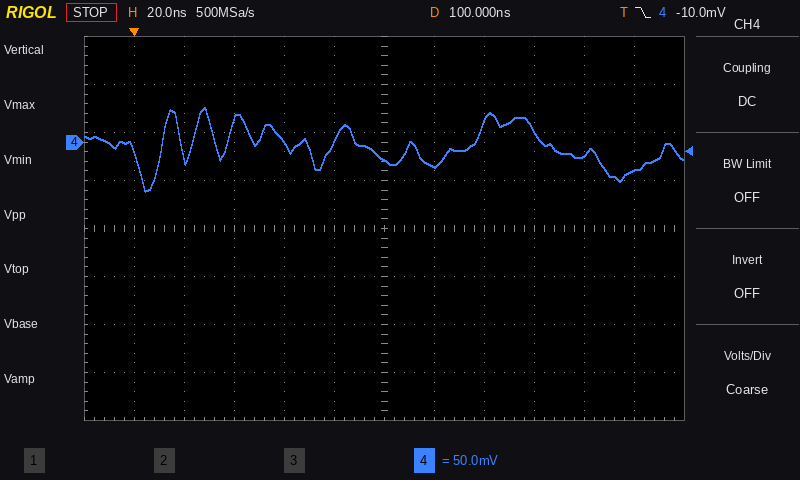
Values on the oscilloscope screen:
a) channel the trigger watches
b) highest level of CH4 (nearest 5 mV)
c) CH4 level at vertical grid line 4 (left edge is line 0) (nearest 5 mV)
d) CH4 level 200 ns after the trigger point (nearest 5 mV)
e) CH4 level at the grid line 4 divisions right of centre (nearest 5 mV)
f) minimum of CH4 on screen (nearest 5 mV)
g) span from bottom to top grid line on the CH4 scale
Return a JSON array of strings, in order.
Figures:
["CH4", "35 mV", "0 mV", "-30 mV", "-15 mV", "-50 mV", "400 mV"]
